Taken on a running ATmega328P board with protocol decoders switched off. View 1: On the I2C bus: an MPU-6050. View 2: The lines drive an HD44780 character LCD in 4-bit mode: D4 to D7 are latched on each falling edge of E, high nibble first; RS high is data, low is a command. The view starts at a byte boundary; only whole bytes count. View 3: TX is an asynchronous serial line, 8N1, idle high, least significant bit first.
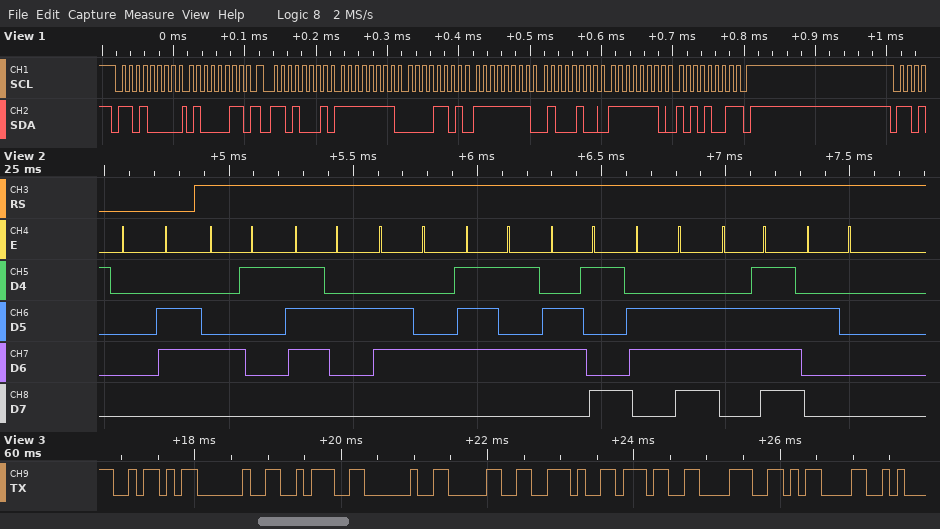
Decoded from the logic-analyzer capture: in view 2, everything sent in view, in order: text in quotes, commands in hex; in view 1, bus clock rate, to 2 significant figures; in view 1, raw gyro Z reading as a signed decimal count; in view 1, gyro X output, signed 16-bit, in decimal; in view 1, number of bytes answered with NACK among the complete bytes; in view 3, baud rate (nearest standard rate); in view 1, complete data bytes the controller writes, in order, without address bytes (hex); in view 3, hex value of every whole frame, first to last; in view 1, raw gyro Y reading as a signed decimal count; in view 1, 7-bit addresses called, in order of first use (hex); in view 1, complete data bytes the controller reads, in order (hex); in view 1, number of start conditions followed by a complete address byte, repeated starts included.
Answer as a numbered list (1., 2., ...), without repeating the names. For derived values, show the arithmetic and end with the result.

1. 0x06 "Arduino "
2. 100 kHz
3. 0xFEA9 = -343
4. 0xFF0D = -243
5. 1
6. 9600 baud
7. 43
8. 5A 20 3A 20 30 2E 37 38 0D
9. 0xFF44 = -188
10. 0x68
11. FF 0D FF 44 FE A9
12. 2
